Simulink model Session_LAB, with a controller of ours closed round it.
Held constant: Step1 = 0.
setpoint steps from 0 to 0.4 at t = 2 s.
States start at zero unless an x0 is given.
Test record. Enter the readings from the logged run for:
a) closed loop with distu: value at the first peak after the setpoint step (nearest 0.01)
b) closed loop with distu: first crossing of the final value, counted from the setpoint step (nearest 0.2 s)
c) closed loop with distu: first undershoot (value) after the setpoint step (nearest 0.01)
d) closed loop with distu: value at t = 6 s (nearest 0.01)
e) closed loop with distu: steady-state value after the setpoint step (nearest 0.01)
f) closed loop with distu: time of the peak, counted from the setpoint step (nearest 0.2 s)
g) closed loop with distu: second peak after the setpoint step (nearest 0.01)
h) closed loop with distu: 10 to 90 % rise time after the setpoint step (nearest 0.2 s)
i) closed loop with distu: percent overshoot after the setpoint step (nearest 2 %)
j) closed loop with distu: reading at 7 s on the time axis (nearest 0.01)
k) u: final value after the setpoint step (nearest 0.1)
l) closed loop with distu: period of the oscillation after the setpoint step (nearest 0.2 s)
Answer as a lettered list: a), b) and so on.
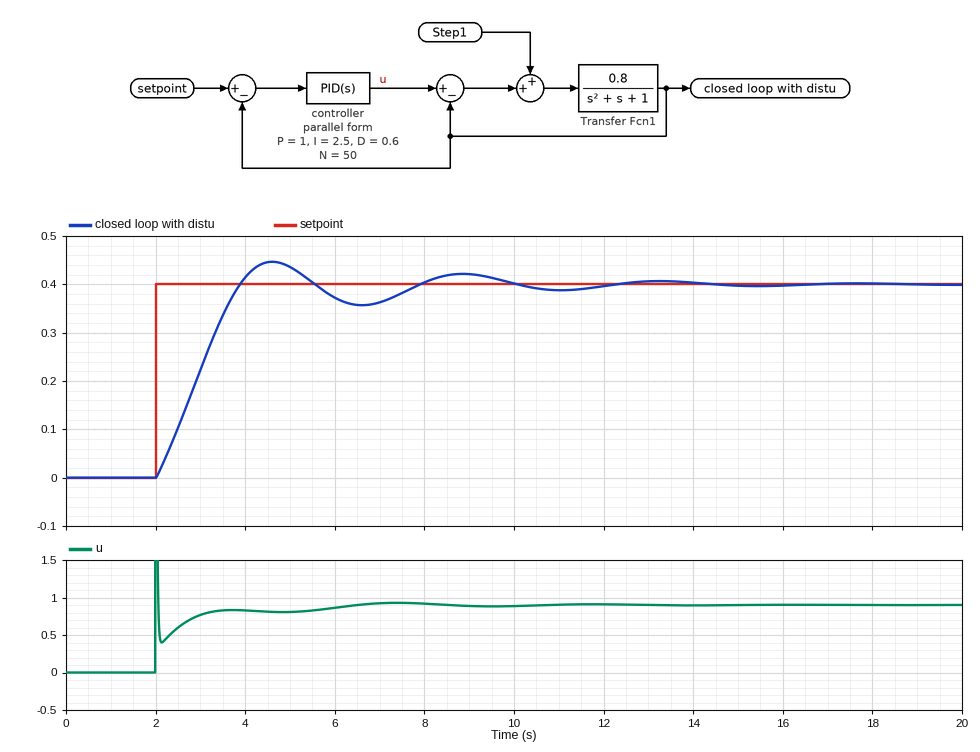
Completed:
a) 0.45
b) 1.8 s
c) 0.36
d) 0.37
e) 0.40
f) 2.6 s
g) 0.42
h) 1.4 s
i) 12 %
j) 0.36
k) 0.9
l) 4.2 s
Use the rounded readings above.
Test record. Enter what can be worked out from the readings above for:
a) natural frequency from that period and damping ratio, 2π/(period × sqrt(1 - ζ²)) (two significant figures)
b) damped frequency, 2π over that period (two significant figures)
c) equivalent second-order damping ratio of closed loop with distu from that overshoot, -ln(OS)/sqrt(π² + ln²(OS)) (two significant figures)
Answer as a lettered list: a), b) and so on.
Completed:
a) 1.8 rad/s
b) 1.5 rad/s
c) 0.56
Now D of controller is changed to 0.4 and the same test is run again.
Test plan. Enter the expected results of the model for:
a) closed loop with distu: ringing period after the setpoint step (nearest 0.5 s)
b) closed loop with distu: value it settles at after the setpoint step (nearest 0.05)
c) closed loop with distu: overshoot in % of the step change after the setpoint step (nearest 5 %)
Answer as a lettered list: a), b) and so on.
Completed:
a) 4.0 s
b) 0.40
c) 20 %
